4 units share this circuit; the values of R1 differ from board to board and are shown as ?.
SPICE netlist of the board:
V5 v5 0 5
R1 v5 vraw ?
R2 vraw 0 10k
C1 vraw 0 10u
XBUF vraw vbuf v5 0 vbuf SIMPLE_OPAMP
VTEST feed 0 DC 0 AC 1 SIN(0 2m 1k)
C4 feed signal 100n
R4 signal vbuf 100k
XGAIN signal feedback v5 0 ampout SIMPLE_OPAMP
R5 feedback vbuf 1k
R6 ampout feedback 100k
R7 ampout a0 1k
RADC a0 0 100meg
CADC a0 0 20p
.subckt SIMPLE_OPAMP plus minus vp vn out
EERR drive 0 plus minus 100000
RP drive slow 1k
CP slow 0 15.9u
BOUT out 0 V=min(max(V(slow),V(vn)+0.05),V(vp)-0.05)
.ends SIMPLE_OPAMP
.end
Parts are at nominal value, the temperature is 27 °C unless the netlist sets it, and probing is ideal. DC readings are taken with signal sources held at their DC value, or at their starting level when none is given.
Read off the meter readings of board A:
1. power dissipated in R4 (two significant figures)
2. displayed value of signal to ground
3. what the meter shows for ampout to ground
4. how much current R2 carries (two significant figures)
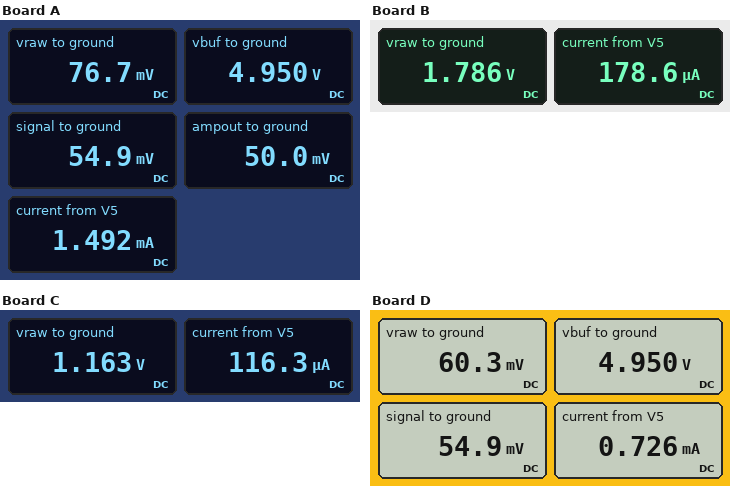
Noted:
240 µW
54.9 mV
50.0 mV
7.7 µA
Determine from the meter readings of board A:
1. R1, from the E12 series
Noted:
3.3 kΩ
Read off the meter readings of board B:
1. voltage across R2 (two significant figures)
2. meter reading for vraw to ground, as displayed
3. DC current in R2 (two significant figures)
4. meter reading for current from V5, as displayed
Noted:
1.8 V
1.786 V
180 µA
178.6 µA
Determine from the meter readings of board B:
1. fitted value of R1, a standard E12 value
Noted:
18 kΩ
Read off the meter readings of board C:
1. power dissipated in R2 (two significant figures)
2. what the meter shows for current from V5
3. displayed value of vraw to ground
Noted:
140 µW
116.3 µA
1.163 V
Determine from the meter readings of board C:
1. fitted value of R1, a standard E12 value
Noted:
33 kΩ
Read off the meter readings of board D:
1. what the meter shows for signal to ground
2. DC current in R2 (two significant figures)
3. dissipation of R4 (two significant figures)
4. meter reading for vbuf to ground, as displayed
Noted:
54.9 mV
6.0 µA
240 µW
4.950 V
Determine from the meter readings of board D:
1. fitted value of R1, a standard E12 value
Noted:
6.8 kΩ
